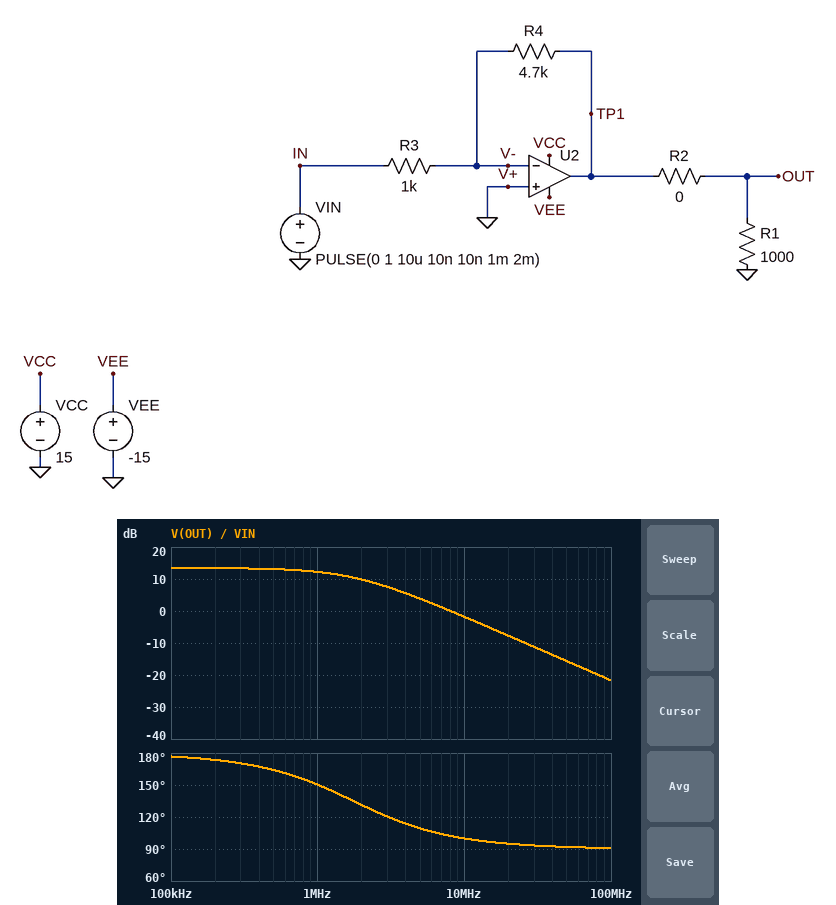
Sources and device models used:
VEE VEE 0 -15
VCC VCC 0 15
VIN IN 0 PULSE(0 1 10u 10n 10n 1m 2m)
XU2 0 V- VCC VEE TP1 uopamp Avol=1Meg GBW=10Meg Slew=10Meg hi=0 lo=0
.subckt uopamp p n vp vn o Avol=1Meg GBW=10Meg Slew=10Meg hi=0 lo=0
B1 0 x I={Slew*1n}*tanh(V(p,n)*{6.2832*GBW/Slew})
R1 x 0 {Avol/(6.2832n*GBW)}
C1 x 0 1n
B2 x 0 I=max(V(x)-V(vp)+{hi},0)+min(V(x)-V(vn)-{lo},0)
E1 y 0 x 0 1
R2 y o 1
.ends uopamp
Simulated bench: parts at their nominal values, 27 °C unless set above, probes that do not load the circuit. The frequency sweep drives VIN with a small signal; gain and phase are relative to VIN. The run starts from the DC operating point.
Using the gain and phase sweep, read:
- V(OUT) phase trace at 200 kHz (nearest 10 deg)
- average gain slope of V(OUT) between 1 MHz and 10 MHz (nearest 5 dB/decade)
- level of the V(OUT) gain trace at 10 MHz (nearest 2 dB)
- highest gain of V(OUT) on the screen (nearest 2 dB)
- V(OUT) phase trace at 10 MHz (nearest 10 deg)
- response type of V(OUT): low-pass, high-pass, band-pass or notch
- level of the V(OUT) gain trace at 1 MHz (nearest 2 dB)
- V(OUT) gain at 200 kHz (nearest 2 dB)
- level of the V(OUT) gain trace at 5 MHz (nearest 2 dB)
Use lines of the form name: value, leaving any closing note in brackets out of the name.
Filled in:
V(OUT) phase trace at 200 kHz: 170 deg
average gain slope of V(OUT) between 1 MHz and 10 MHz: -15 dB/decade
level of the V(OUT) gain trace at 10 MHz: -2 dB
highest gain of V(OUT) on the screen: 14 dB
V(OUT) phase trace at 10 MHz: 100 deg
response type of V(OUT): low-pass, high-pass, band-pass or notch: low-pass
level of the V(OUT) gain trace at 1 MHz: 12 dB
V(OUT) gain at 200 kHz: 14 dB
level of the V(OUT) gain trace at 5 MHz: 4 dB
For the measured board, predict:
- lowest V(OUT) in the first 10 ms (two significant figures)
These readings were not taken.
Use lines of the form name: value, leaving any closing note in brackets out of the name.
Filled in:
lowest V(OUT) in the first 10 ms: -4.7 V
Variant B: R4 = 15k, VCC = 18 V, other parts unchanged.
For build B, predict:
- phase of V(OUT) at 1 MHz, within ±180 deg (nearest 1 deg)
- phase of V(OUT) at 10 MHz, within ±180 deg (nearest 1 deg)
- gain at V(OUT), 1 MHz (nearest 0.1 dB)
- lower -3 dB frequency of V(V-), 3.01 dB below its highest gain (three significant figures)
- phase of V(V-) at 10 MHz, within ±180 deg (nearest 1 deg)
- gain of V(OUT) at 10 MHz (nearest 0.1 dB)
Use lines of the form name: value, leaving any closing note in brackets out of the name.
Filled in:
phase of V(OUT) at 1 MHz, within ±180 deg: 122 deg
phase of V(OUT) at 10 MHz, within ±180 deg: 94 deg
gain at V(OUT), 1 MHz: 18.0 dB
lower -3 dB frequency of V(V-), 3.01 dB below its highest gain: 624 kHz
phase of V(V-) at 10 MHz, within ±180 deg: 4 deg
gain of V(OUT) at 10 MHz: -0.6 dB
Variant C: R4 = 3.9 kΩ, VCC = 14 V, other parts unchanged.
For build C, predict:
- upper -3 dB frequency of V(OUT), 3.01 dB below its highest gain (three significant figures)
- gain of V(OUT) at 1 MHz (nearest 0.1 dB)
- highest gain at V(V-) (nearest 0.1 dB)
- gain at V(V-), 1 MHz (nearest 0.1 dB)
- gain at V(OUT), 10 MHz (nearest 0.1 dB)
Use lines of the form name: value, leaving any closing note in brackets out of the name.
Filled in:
upper -3 dB frequency of V(OUT), 3.01 dB below its highest gain: 2.04 MHz
gain of V(OUT) at 1 MHz: 10.9 dB
highest gain at V(V-): -2.0 dB
gain at V(V-), 1 MHz: -9.1 dB
gain at V(OUT), 10 MHz: -2.2 dB
